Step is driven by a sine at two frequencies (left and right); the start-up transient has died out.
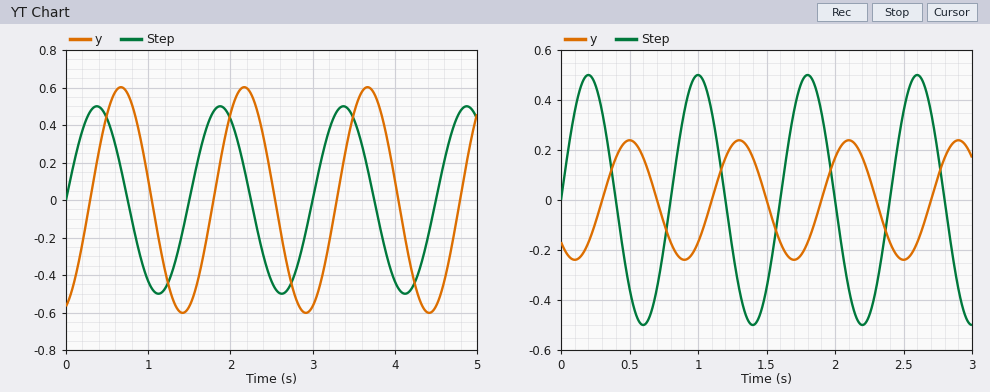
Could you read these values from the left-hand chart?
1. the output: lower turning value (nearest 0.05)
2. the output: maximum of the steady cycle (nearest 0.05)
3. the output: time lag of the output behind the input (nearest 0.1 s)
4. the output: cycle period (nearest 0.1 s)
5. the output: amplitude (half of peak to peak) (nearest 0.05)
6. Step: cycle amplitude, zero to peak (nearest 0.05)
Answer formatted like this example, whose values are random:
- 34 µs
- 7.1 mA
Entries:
- -0.60
- 0.60
- 0.3 s
- 1.5 s
- 0.60
- 0.50
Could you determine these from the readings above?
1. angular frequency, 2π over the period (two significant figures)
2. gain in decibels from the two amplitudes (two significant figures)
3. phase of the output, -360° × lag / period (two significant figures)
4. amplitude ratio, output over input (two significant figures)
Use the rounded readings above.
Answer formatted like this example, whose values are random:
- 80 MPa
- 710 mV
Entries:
- 4.2 rad/s
- 1.6 dB
- -72°
- 1.2
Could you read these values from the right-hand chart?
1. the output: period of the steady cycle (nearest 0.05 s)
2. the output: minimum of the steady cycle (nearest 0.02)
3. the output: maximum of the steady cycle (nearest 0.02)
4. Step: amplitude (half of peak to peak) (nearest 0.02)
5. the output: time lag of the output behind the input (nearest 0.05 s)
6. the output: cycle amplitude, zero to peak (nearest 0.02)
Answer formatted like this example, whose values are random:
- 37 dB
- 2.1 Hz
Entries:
- 0.80 s
- -0.24
- 0.24
- 0.50
- 0.30 s
- 0.24
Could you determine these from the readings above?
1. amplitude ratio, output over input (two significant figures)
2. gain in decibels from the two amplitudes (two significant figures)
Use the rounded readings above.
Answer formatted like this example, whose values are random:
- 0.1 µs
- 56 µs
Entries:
- 0.48
- -6.4 dB
